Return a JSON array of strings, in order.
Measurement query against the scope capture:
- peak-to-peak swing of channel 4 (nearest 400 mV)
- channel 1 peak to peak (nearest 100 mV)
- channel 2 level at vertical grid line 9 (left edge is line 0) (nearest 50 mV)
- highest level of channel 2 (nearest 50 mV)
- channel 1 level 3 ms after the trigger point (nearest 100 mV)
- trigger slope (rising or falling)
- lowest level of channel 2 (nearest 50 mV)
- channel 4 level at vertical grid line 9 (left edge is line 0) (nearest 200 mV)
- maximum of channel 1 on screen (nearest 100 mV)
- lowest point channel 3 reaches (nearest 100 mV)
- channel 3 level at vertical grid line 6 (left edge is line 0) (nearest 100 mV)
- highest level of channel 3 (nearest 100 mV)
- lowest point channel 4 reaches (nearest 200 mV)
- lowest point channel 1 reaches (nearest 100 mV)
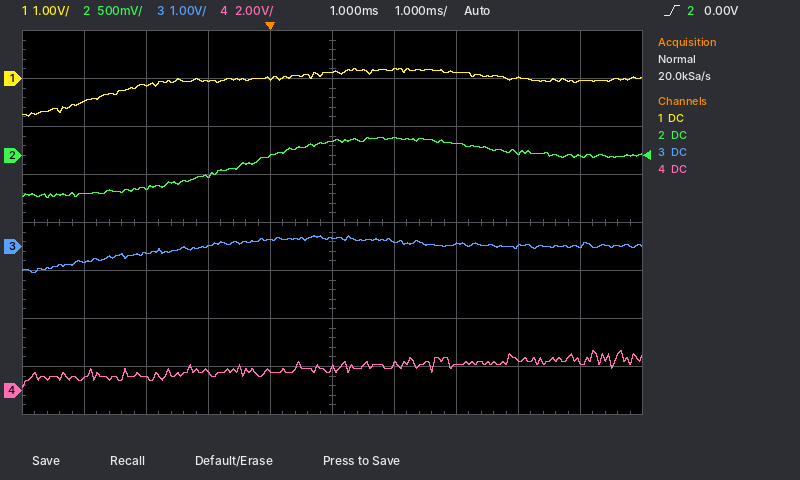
["1.6 V", "1.0 V", "0 mV", "200 mV", "100 mV", "rising", "-450 mV", "1.2 V", "200 mV", "-500 mV", "100 mV", "200 mV", "200 mV", "-800 mV"]
